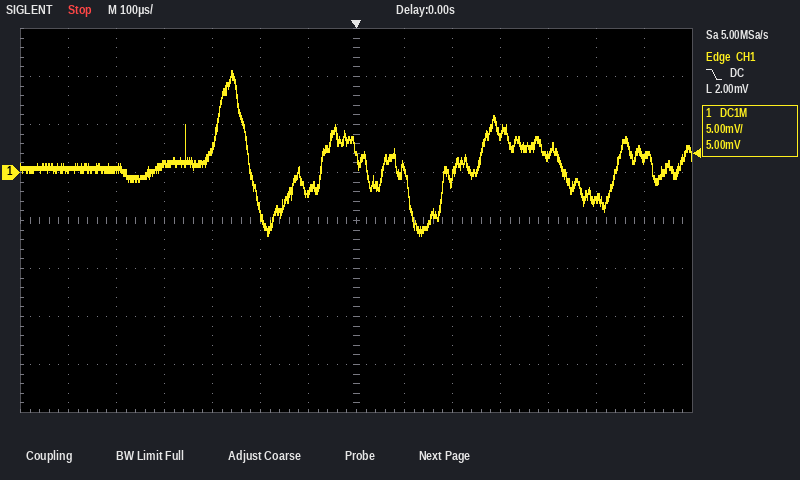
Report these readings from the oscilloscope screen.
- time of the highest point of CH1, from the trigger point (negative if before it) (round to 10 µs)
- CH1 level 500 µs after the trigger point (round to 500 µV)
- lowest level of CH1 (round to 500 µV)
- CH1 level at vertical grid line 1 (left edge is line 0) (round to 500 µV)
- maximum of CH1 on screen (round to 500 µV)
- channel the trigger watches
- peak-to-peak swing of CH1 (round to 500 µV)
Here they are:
-260 µs
-2.5 mV
-6.5 mV
500 µV
10.5 mV
CH1
17.0 mV
